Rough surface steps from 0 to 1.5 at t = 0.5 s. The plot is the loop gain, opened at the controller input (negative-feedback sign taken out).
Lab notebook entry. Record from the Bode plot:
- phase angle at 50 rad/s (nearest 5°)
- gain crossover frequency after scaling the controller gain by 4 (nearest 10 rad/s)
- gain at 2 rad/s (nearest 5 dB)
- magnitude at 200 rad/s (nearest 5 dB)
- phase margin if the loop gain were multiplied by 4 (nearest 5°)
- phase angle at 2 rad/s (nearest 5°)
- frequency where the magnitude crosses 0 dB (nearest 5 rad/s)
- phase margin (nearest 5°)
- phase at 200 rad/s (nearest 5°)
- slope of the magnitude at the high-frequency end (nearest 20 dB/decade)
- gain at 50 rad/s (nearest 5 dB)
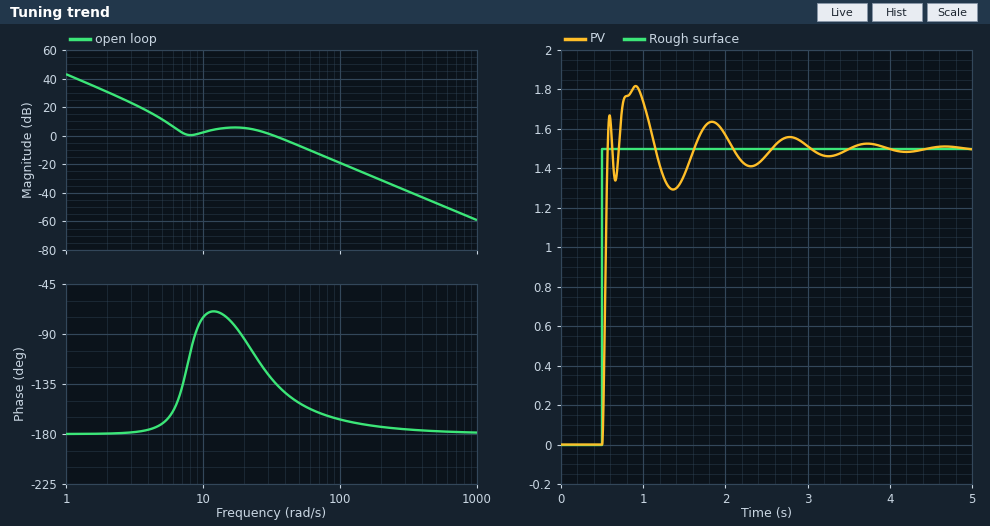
-150°
70 rad/s
30 dB
-30 dB
20°
-180°
35 rad/s
45°
-175°
-40 dB/decade
-5 dB
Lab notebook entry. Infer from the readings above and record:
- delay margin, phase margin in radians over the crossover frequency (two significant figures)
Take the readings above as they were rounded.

0.022 s
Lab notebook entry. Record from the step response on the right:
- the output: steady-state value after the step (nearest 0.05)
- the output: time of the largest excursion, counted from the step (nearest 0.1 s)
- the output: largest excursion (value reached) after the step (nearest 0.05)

1.50
0.4 s
1.80
